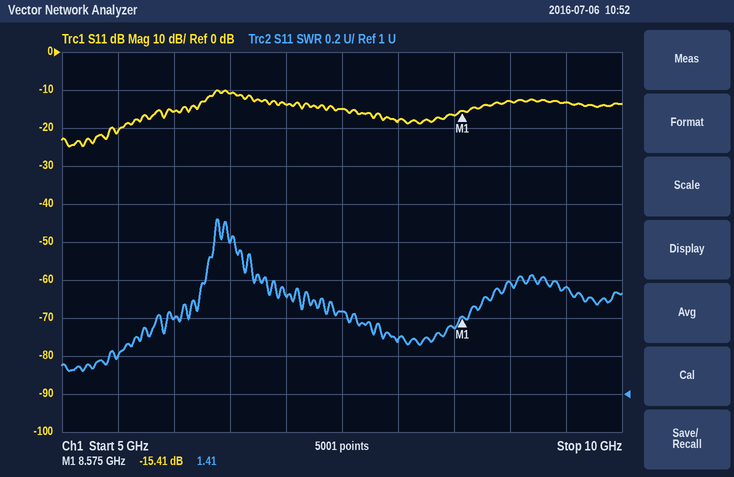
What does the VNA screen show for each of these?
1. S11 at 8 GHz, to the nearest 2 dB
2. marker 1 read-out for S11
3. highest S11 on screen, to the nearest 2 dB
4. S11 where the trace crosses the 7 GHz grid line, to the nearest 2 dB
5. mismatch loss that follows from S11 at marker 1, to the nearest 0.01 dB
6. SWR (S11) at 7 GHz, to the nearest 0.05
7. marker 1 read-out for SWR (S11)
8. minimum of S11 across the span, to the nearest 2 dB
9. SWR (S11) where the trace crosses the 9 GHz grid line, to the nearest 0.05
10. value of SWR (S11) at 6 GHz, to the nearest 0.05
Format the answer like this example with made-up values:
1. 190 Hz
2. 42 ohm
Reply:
1. -18 dB
2. -15.41 dB
3. -10 dB
4. -14 dB
5. 0.13 dB
6. 1.50
7. 1.41
8. -24 dB
9. 1.60
10. 1.40
